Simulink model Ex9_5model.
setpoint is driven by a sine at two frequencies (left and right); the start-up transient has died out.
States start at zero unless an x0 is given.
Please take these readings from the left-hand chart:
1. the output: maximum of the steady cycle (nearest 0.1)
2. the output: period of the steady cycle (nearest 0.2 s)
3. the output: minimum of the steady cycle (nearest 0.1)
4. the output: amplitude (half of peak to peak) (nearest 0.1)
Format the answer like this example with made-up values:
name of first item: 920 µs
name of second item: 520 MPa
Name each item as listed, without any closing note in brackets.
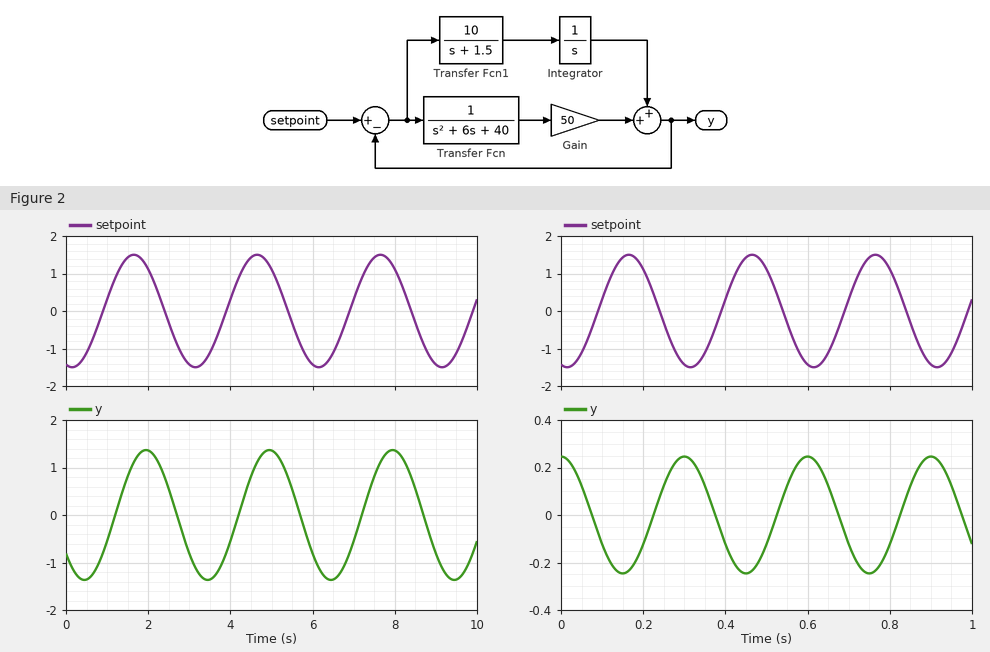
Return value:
the output: maximum of the steady cycle: 1.4
the output: period of the steady cycle: 3.0 s
the output: minimum of the steady cycle: -1.4
the output: amplitude (half of peak to peak): 1.4
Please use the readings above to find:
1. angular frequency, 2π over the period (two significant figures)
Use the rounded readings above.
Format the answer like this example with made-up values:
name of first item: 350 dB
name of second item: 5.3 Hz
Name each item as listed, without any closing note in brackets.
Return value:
angular frequency, 2π over the period: 2.1 rad/s
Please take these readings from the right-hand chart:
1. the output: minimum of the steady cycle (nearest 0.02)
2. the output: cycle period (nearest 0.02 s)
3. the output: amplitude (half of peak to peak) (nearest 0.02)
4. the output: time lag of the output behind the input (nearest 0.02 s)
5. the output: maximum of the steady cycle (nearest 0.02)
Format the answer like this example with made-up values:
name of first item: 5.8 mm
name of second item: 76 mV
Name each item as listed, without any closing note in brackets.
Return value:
the output: minimum of the steady cycle: -0.24
the output: cycle period: 0.30 s
the output: amplitude (half of peak to peak): 0.24
the output: time lag of the output behind the input: 0.14 s
the output: maximum of the steady cycle: 0.24
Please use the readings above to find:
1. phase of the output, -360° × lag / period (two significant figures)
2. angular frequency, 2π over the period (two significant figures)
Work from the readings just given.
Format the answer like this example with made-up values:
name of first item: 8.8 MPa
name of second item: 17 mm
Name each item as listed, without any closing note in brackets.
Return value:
phase of the output, -360° × lag / period: -170°
angular frequency, 2π over the period: 21 rad/s
